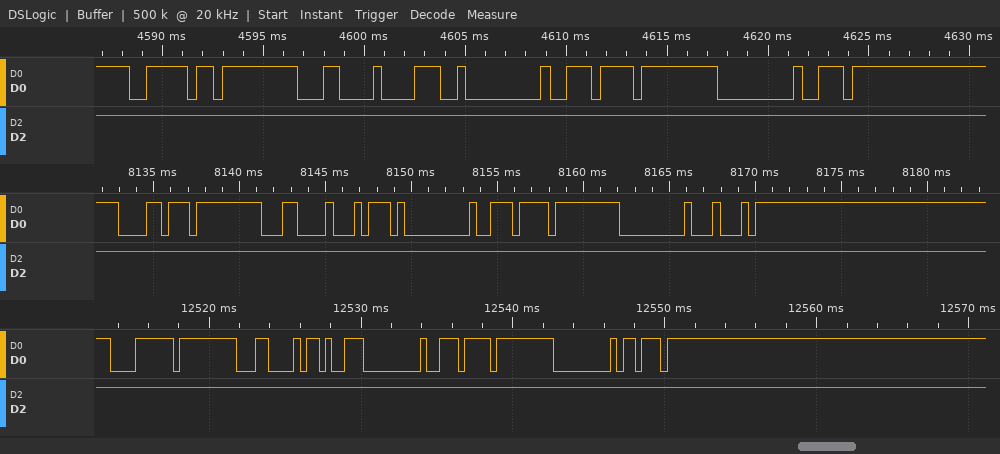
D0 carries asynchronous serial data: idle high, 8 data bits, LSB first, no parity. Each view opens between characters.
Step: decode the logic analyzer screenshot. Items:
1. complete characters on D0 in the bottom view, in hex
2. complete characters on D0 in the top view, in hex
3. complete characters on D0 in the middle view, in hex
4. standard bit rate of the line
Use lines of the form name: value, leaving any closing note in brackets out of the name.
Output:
complete characters on D0 in the bottom view, in hex: F8, FF, 0C, CB, 00, EE, FF, 00, BB
complete characters on D0 in the top view, in hex: BE, FF, 0C, 38, 00, EE, FF, 00, EE
complete characters on D0 in the middle view, in hex: D8, FF, 0C, 74, 00, EE, FF, 00, 44
standard bit rate of the line: 2400 baud
